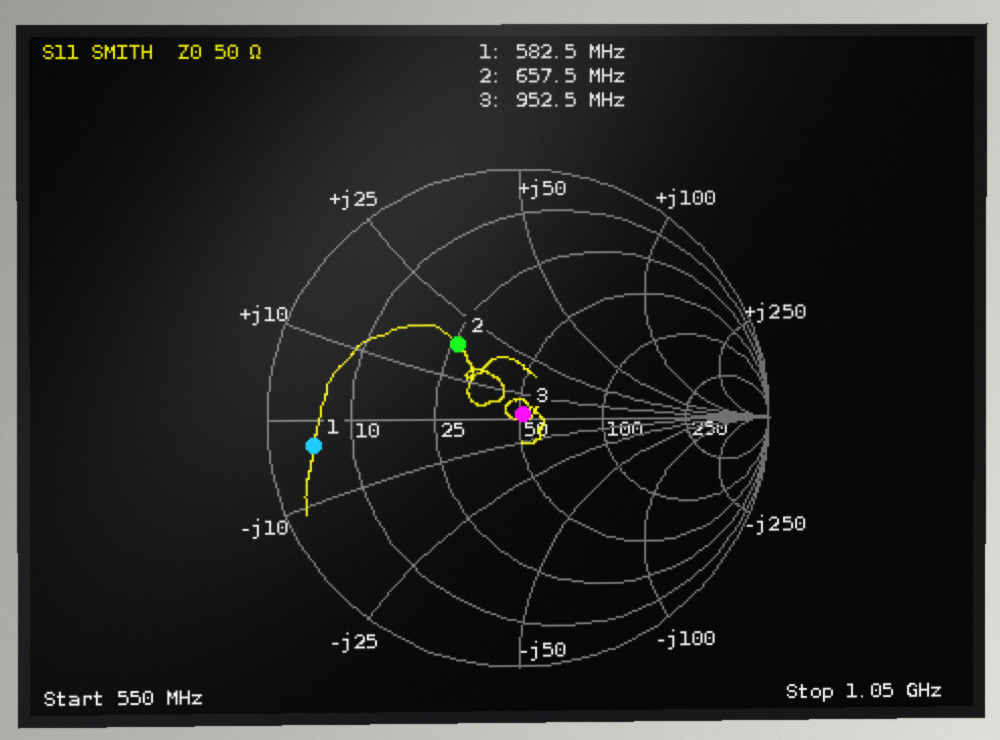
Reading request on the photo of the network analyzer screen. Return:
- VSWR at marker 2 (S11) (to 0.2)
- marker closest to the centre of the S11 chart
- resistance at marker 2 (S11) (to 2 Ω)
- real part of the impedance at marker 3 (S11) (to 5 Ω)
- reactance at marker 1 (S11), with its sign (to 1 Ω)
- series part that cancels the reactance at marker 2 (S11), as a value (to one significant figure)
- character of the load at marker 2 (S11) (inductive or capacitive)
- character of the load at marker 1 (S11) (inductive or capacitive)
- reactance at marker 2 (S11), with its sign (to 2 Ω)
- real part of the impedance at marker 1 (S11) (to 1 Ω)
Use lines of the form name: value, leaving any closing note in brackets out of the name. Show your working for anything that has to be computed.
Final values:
VSWR at marker 2 (S11): 2.2
marker closest to the centre of the S11 chart: marker 3
resistance at marker 2 (S11): 26 Ω
real part of the impedance at marker 3 (S11): 50 Ω
reactance at marker 1 (S11), with its sign: -3 Ω
series part that cancels the reactance at marker 2 (S11), as a value: C = 1/(2π × 657.5 MHz × 18 Ω) ≈ 13.4 pF, so 10 pF to one significant figure
character of the load at marker 2 (S11): inductive
character of the load at marker 1 (S11): capacitive
reactance at marker 2 (S11), with its sign: +18 Ω
real part of the impedance at marker 1 (S11): 5 Ω
